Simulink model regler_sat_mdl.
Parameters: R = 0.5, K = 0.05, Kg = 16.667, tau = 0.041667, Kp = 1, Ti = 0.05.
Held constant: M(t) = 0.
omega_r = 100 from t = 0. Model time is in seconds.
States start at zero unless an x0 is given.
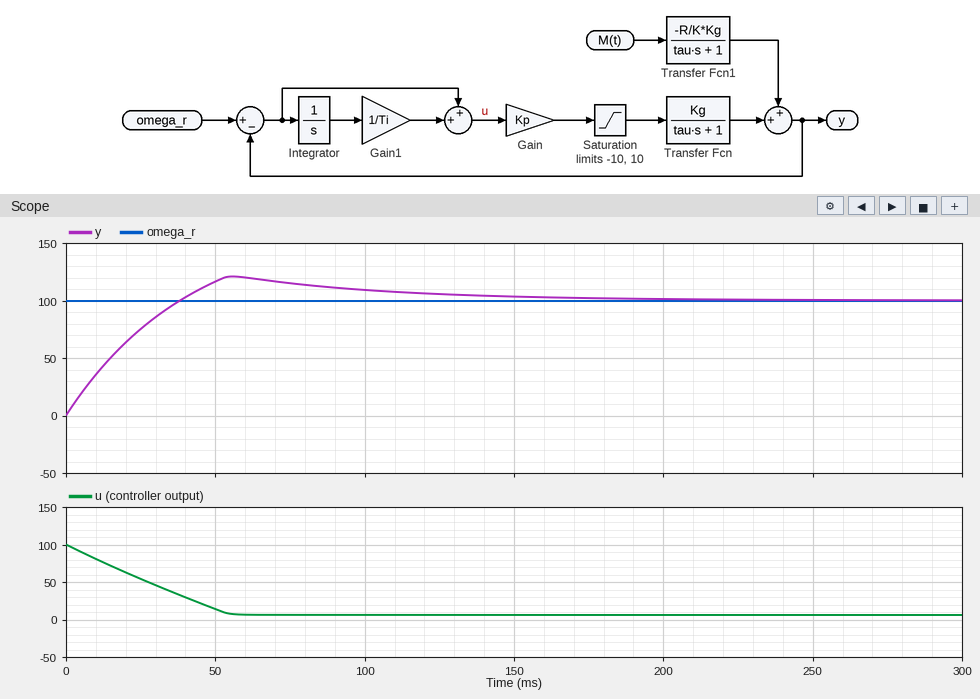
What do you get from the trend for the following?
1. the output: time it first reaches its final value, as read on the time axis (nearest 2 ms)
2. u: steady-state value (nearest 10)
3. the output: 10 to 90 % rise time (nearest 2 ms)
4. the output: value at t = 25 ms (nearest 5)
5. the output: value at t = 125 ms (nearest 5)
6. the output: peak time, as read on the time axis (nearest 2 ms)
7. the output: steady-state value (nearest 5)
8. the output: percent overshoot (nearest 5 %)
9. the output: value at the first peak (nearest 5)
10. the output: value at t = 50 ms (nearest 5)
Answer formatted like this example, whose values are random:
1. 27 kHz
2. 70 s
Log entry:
1. 38 ms
2. 10
3. 30 ms
4. 75
5. 105
6. 56 ms
7. 100
8. 20 %
9. 120
10. 115
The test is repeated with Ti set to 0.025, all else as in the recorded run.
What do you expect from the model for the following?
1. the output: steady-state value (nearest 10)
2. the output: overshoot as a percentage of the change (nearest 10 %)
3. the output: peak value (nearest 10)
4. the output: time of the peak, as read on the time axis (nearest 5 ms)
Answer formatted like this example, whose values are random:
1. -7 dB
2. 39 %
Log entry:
1. 100
2. 30 %
3. 130
4. 70 ms
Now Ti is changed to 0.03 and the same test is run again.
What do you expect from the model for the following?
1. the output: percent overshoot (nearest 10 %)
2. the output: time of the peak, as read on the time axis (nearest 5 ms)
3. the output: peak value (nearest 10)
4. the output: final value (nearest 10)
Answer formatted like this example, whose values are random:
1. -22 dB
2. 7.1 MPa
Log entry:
1. 30 %
2. 65 ms
3. 130
4. 100
